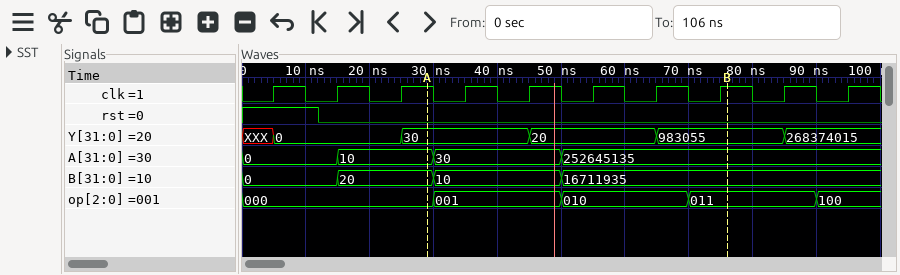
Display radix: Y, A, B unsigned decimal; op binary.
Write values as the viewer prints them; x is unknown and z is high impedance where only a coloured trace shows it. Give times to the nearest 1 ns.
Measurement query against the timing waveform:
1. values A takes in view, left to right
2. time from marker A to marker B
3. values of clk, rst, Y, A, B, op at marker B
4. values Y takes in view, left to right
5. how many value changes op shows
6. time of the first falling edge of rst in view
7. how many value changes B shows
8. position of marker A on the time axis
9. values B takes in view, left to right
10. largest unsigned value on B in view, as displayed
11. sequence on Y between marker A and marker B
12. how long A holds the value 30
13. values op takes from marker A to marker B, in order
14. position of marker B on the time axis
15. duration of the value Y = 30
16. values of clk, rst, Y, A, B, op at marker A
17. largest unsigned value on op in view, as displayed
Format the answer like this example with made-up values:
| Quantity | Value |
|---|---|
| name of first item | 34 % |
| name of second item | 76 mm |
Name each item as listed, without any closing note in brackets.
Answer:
| Quantity | Value |
|---|---|
| values A takes in view, left to right | 0, 10, 30, 252645135 |
| time from marker A to marker B | 47 ns |
| values of clk, rst, Y, A, B, op at marker B | clk=1, rst=0, Y=983055, A=252645135, B=16711935, op=011 |
| values Y takes in view, left to right | XXX, 0, 30, 20, 983055, 268374015 |
| how many value changes op shows | 4 |
| time of the first falling edge of rst in view | 12 ns |
| how many value changes B shows | 3 |
| position of marker A on the time axis | 29 ns |
| values B takes in view, left to right | 0, 20, 10, 16711935 |
| largest unsigned value on B in view, as displayed | 16711935 |
| sequence on Y between marker A and marker B | 30, 20, 983055 |
| how long A holds the value 30 | 20 ns |
| values op takes from marker A to marker B, in order | 000, 001, 010, 011 |
| position of marker B on the time axis | 76 ns |
| duration of the value Y = 30 | 20 ns |
| values of clk, rst, Y, A, B, op at marker A | clk=1, rst=0, Y=30, A=10, B=20, op=000 |
| largest unsigned value on op in view, as displayed | 100 |
